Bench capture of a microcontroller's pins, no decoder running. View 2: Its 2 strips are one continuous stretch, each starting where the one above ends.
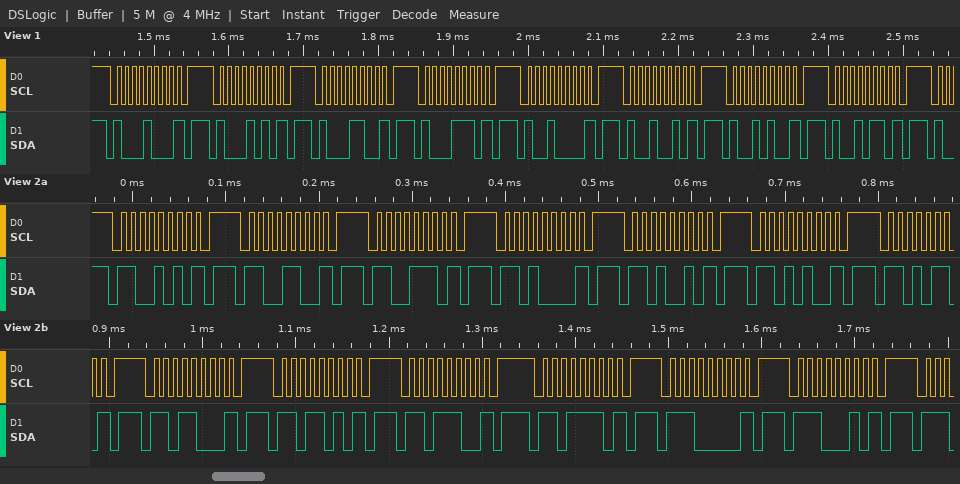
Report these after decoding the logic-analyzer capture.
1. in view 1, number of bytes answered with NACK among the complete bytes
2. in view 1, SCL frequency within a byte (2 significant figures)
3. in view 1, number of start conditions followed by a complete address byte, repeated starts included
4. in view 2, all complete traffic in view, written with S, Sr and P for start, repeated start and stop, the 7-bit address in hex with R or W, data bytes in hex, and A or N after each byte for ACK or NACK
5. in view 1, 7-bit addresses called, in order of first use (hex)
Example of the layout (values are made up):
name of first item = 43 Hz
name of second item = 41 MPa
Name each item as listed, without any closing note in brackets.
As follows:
in view 1, number of bytes answered with NACK among the complete bytes = 8
in view 1, SCL frequency within a byte = 100 kHz
in view 1, number of start conditions followed by a complete address byte, repeated starts included = 8
in view 2, all complete traffic in view, written with S, Sr and P for start, repeated start and stop, the 7-bit address in hex with R or W, data bytes in hex, and A or N after each byte for ACK or NACK = S 65W N P S 66W N P S 67W N P S 68W N P S 69W N P S 6AW N P S 6BW N P S 6CW N P S 6DW N P S 6EW N P S 6FW N P S 70W N P S 71W N P
in view 1, 7-bit addresses called, in order of first use = 0x44 0x45 0x46 0x47 0x48 0x49 0x4A 0x4B
